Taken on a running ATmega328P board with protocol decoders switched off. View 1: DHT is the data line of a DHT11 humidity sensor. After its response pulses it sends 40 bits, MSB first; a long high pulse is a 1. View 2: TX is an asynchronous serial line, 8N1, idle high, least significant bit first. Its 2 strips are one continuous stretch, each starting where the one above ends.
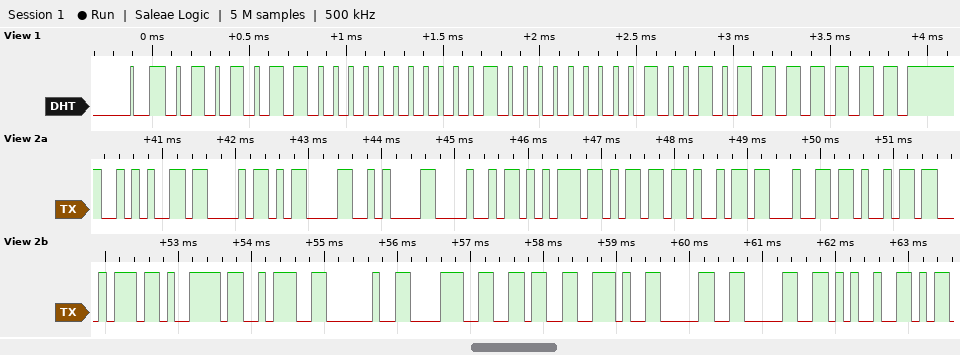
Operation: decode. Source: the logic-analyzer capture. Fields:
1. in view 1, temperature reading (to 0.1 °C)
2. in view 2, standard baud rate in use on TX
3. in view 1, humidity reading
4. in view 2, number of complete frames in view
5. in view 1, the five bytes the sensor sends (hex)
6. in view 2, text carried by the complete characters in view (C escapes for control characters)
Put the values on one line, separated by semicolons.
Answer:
32.9 °C; 9600 baud; 86 %; 20; 56 00 20 09 7F; "*C\r\nHumidity: 86.00%"
